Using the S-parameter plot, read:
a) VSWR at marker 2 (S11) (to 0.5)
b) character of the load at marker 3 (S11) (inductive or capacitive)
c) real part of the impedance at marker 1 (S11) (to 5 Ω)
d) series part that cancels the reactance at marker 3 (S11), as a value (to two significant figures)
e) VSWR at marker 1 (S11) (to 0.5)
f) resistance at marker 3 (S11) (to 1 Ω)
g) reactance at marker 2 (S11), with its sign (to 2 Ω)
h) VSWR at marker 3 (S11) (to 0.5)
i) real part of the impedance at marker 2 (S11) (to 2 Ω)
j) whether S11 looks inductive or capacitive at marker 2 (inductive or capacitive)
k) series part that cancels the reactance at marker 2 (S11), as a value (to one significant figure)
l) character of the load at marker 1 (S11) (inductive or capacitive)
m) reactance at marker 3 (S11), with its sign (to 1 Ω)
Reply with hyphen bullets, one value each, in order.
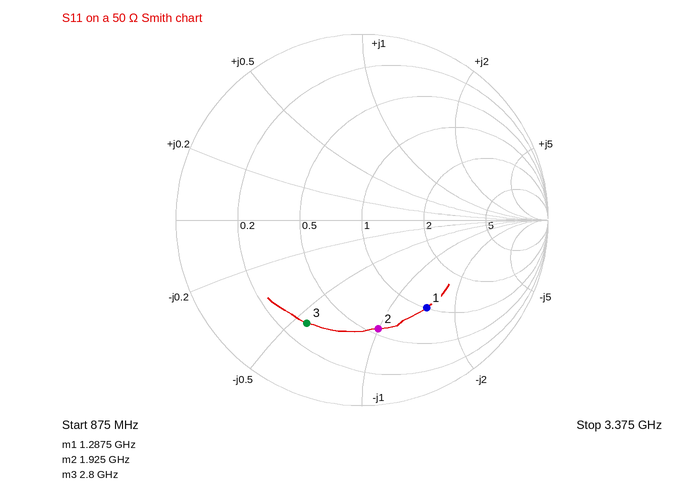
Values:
- 4.0
- capacitive
- 50 Ω
- 1.6 nH
- 4.0
- 15 Ω
- -50 Ω
- 4.5
- 28 Ω
- capacitive
- 4 nH
- capacitive
- -28 Ω
